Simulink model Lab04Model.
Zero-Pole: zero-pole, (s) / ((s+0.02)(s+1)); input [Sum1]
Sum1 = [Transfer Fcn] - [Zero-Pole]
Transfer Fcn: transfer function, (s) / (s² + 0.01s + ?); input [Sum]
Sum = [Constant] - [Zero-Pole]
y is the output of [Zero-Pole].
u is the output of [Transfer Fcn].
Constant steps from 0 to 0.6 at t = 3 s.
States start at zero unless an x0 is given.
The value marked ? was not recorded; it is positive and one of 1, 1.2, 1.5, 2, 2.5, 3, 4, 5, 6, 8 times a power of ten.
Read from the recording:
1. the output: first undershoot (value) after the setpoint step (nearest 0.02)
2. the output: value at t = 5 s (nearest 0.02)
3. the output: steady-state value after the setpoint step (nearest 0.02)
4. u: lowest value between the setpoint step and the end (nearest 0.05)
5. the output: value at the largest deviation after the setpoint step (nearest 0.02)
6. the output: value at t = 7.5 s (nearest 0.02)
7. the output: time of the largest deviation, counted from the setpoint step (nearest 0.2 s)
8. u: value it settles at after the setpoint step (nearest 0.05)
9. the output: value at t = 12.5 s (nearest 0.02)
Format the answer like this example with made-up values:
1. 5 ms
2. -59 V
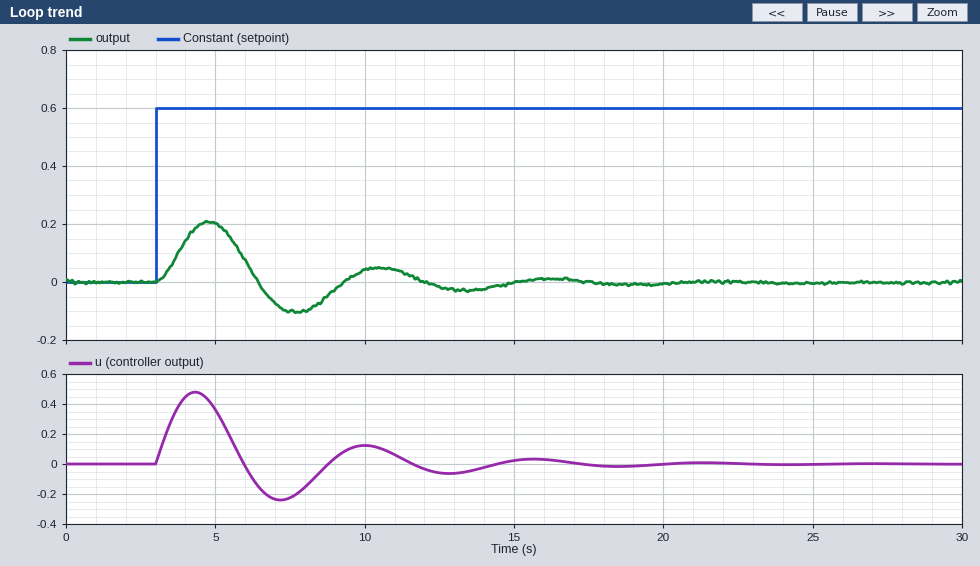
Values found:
1. -0.10
2. 0.20
3. 0.00
4. -0.25
5. 0.20
6. -0.10
7. 1.8 s
8. 0.00
9. -0.02
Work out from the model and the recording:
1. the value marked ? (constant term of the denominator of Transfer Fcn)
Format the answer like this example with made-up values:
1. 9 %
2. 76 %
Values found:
1. 1
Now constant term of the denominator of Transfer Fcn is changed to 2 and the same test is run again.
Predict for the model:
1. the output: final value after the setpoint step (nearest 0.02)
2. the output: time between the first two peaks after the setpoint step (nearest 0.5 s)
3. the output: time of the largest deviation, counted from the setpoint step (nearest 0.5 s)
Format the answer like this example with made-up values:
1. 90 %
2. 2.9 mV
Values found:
1. 0.00
2. 4.0 s
3. 1.5 s
